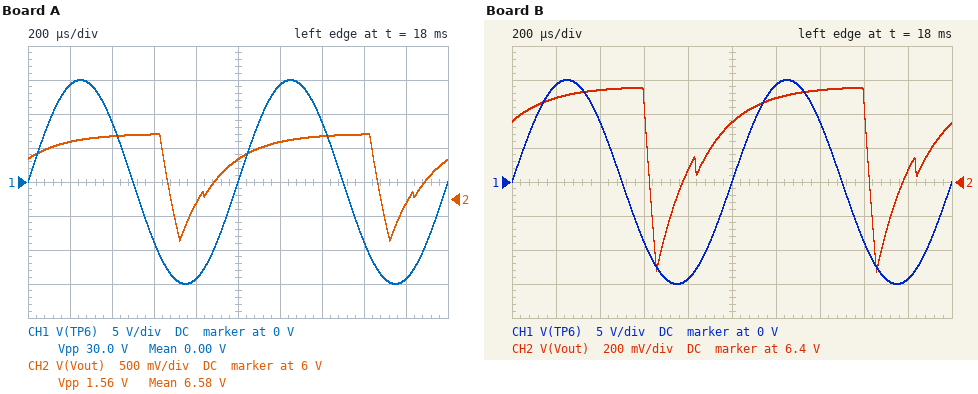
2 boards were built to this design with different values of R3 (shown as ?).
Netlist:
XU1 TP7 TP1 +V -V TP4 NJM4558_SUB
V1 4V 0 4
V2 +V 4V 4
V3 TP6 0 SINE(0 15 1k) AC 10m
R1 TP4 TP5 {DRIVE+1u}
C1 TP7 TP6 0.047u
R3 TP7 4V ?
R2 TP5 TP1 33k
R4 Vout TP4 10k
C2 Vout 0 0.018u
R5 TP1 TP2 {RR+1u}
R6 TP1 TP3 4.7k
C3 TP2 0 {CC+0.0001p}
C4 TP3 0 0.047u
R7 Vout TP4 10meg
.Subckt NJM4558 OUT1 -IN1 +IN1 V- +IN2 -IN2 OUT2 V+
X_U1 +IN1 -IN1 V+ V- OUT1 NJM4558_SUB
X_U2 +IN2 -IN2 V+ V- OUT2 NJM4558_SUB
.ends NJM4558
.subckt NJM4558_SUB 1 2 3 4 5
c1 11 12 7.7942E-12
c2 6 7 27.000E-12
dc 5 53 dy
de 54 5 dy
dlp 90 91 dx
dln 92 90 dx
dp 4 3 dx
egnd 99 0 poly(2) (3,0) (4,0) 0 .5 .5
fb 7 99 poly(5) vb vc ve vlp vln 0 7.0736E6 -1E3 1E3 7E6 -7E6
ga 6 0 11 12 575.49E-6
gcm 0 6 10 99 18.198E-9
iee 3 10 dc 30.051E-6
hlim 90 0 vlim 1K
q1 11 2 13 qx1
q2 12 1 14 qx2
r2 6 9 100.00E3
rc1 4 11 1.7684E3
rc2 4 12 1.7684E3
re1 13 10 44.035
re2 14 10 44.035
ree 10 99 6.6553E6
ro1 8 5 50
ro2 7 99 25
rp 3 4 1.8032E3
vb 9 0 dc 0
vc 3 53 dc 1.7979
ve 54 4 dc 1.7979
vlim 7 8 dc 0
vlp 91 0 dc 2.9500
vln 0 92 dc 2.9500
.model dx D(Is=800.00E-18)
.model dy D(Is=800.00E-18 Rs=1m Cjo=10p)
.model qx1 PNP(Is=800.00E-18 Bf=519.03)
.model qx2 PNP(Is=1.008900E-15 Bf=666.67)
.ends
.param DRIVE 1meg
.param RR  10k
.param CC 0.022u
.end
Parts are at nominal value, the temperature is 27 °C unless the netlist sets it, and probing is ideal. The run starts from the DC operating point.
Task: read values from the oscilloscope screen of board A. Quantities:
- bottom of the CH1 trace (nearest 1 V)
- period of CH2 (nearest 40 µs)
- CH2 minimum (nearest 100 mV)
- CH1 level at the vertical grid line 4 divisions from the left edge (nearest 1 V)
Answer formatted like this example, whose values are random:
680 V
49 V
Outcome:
-15 V
1.00 ms
5.4 V
-14 V
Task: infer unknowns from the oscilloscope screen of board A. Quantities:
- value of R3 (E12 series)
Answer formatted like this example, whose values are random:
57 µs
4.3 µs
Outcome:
120 kΩ
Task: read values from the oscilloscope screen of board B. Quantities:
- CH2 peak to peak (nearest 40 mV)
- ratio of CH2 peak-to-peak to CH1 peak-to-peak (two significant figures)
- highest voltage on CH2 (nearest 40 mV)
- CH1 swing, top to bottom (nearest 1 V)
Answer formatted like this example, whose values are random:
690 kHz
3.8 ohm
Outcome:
1.08 V
0.036
6.96 V
30 V
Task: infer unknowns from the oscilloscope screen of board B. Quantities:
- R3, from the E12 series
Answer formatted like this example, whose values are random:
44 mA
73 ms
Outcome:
56 kΩ
